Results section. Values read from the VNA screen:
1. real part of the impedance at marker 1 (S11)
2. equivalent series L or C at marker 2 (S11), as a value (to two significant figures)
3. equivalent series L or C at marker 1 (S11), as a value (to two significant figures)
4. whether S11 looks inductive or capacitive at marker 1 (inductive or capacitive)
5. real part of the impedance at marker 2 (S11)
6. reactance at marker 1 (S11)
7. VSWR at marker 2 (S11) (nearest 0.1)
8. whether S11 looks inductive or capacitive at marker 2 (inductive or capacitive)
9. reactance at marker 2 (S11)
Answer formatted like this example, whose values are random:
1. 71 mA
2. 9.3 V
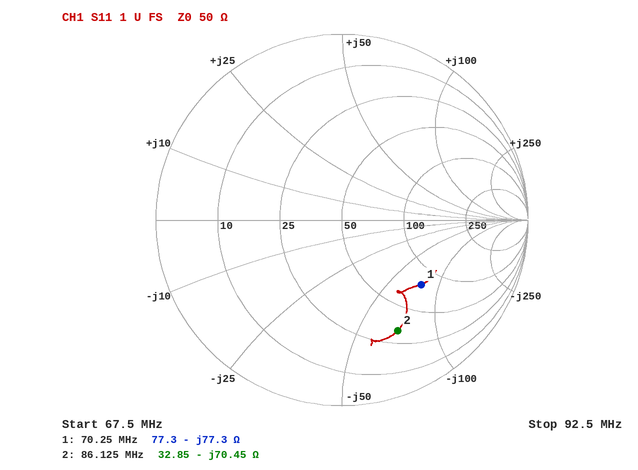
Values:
1. 77.3 Ω
2. 26 pF
3. 29 pF
4. capacitive
5. 32.85 Ω
6. -77.3 Ω
7. 5.0
8. capacitive
9. -70.45 Ω
